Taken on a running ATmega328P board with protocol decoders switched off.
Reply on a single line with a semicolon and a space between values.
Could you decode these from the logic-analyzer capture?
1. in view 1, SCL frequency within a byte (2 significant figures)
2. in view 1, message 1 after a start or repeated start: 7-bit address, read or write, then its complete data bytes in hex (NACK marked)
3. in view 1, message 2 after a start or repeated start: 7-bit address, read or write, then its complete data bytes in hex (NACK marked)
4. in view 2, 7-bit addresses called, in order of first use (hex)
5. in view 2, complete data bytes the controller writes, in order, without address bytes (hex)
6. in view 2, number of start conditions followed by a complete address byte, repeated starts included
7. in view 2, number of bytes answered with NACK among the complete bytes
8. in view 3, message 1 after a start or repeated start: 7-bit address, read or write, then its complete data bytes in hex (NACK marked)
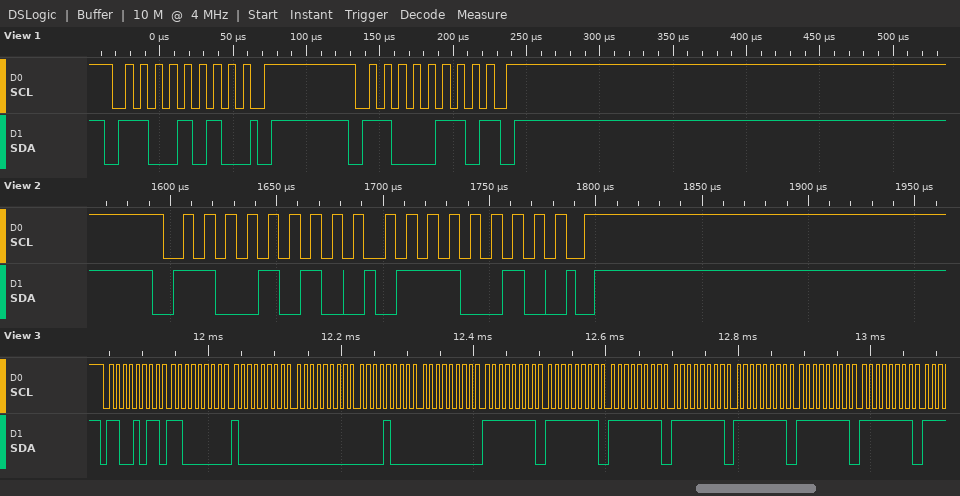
100 kHz; 0x65 write; 0x63 write NACK; 0x65; 72; 1; 0; 0x65 read: C0 80 00 08 00 FF FF FF FF FF FF FF
